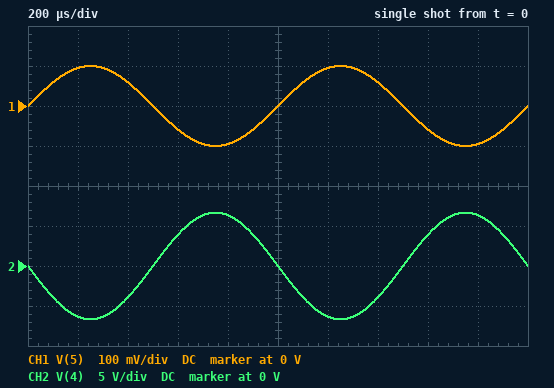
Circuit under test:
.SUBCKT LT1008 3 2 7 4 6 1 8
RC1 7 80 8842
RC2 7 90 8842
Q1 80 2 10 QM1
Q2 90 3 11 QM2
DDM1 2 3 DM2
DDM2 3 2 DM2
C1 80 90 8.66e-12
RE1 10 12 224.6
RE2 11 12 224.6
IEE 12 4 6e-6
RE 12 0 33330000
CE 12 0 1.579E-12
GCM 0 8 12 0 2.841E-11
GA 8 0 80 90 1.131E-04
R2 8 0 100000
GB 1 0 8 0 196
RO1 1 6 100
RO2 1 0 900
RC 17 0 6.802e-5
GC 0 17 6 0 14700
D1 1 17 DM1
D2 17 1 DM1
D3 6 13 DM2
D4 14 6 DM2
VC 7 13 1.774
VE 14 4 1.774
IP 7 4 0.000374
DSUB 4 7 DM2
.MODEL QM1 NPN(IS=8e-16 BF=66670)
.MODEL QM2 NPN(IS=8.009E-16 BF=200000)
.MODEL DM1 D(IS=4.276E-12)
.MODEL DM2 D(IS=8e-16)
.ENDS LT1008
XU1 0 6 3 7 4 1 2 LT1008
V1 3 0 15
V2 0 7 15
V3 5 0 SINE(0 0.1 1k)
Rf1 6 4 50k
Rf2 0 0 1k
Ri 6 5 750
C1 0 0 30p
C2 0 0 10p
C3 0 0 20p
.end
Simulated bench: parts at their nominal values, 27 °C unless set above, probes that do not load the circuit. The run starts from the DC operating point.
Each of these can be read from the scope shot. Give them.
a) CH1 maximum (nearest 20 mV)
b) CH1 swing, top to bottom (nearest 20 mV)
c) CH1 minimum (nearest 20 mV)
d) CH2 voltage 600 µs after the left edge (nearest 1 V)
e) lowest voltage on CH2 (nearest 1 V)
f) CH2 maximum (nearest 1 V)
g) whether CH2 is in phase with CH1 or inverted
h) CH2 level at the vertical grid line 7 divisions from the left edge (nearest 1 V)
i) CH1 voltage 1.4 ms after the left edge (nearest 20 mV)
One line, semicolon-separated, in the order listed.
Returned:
100 mV; 200 mV; -100 mV; 4 V; -7 V; 7 V; inverted; -4 V; 60 mV
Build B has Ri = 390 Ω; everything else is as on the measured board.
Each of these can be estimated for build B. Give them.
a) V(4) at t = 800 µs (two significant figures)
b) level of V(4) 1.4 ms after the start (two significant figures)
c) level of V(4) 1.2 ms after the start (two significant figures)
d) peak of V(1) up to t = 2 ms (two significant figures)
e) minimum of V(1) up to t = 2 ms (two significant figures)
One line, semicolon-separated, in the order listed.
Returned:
12 V; -7.5 V; -12 V; 13 V; -13 V
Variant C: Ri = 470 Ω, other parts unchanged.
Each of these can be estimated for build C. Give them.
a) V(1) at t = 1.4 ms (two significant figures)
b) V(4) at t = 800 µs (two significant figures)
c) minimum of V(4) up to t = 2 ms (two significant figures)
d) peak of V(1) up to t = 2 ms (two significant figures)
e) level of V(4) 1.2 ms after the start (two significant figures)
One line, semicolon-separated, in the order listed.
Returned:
-6.3 V; 10 V; -11 V; 11 V; -10 V
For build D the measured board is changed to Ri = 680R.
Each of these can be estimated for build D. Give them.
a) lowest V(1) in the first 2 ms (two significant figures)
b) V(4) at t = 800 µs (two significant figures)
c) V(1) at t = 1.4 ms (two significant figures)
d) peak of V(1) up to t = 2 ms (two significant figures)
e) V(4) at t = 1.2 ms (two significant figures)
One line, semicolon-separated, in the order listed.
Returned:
-7.4 V; 7.0 V; -4.3 V; 7.4 V; -7.0 V
